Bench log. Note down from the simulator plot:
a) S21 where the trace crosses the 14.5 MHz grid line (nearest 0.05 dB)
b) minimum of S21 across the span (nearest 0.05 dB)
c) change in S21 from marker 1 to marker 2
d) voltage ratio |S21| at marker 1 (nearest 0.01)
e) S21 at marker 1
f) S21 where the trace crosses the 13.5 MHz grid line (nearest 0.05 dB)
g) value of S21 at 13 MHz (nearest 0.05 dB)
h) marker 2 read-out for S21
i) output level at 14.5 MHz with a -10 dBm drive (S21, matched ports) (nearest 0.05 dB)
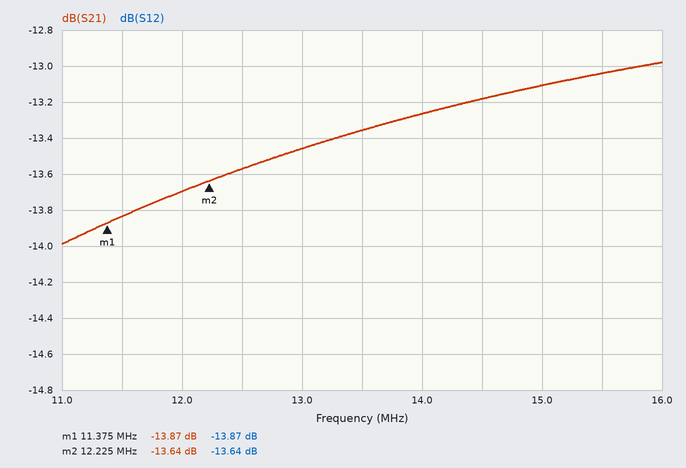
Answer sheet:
-13.20 dB
-14.00 dB
0.23 dB
0.20
-13.87 dB
-13.35 dB
-13.45 dB
-13.64 dB
-23.20 dBm
